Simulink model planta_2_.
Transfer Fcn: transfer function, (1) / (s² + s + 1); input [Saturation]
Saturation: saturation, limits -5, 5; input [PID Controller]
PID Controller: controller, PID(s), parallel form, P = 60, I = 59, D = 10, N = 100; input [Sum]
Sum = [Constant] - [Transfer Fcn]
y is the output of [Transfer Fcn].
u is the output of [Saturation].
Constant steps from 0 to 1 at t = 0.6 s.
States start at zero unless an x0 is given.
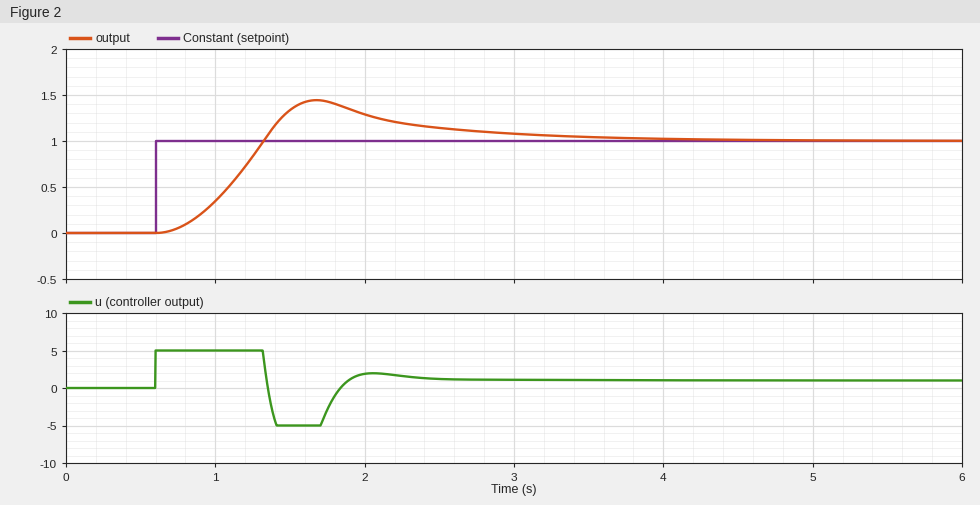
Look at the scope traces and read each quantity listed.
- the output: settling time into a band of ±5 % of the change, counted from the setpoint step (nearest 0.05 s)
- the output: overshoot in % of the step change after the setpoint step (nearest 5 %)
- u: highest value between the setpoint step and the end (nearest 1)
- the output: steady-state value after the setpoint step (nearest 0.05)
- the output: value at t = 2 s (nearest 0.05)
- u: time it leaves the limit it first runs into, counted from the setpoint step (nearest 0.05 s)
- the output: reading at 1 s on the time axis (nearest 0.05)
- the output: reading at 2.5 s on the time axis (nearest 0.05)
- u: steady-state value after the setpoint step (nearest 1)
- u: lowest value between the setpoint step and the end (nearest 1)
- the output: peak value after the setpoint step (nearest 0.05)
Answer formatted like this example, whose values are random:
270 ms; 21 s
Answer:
2.80 s; 45 %; 5; 1.00; 1.30; 0.70 s; 0.35; 1.15; 1; -5; 1.45
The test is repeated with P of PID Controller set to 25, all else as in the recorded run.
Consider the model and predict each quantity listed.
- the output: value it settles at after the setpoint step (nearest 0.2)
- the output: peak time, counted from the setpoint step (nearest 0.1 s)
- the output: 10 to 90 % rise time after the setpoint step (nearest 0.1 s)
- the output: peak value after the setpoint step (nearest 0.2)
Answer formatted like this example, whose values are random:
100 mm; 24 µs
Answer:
1.0; 1.2 s; 0.5 s; 1.6
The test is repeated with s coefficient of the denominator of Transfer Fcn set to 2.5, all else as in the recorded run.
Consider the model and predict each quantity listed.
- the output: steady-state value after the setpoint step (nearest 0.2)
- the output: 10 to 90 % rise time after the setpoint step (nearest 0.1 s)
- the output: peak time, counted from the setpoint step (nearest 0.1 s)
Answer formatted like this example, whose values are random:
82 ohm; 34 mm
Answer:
1.0; 0.6 s; 1.3 s
